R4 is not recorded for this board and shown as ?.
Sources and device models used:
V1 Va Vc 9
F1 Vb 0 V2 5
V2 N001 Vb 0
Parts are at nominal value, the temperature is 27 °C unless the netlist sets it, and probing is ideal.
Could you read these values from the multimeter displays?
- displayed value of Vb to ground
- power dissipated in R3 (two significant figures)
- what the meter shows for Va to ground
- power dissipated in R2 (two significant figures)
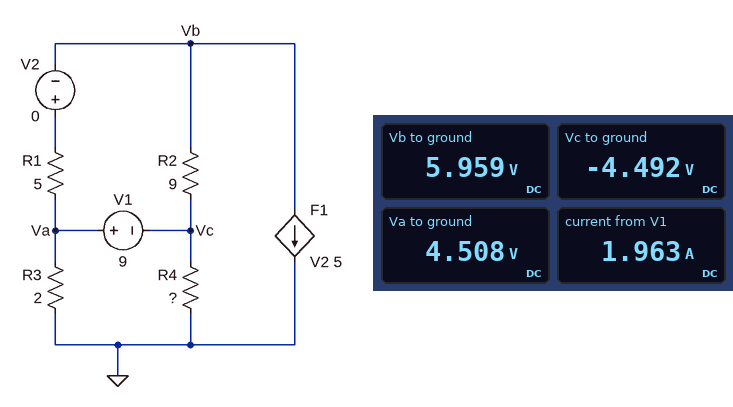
5.959 V
10 W
4.508 V
12 W
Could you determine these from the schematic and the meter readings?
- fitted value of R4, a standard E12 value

5.6 Ω
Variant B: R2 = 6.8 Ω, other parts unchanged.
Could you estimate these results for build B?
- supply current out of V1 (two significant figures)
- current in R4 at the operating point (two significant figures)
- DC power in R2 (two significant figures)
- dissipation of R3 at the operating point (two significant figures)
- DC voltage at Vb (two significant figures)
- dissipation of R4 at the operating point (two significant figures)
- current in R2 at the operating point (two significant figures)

2.3 A
650 mA
18 W
14 W
7.4 V
2.4 W
1.6 A
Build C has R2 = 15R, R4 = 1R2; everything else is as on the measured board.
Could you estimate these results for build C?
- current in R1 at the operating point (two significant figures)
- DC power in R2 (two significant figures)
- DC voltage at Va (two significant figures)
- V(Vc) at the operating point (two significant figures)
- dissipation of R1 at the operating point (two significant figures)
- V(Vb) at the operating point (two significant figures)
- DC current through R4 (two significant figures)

160 mA
6.4 W
6.2 V
-2.8 V
130 mW
7.1 V
2.3 A
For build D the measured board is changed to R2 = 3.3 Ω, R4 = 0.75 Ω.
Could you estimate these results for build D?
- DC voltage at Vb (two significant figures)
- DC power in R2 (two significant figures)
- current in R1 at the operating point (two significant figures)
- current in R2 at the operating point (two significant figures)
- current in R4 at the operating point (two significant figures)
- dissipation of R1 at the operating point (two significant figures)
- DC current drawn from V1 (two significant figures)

15 V
64 W
1.1 A
4.4 A
720 mA
6.0 W
3.7 A
